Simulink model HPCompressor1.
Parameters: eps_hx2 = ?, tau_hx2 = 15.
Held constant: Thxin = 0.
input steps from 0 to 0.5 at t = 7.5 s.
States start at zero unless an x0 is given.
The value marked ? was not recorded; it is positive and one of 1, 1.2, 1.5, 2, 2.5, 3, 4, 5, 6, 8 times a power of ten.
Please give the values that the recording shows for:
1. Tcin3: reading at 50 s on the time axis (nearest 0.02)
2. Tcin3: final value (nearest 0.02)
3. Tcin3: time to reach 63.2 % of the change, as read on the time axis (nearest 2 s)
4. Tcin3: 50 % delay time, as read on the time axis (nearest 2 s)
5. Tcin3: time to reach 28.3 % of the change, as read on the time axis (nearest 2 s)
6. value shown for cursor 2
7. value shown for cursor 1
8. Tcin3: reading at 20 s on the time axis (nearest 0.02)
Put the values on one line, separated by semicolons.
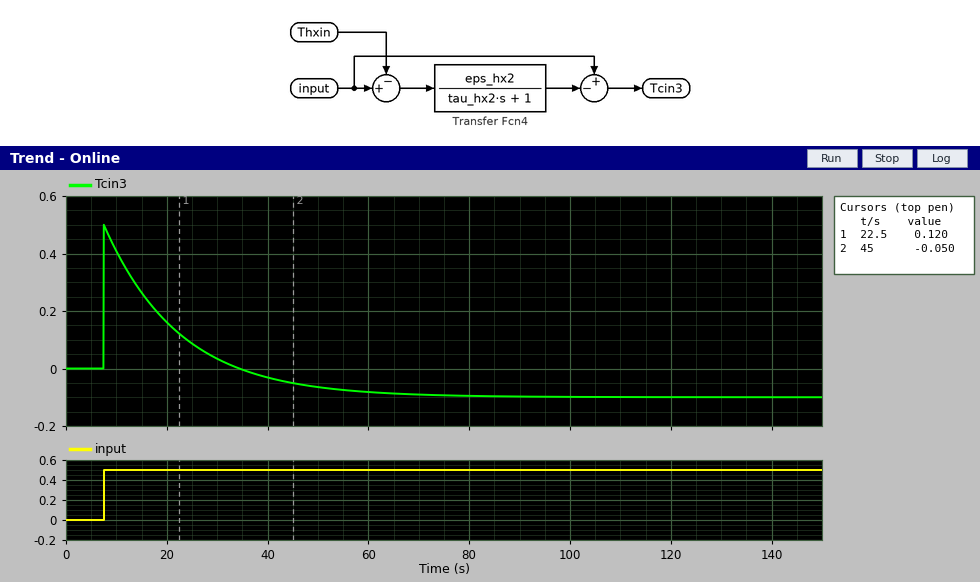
-0.06; -0.10; 50 s; 44 s; 40 s; -0.050; 0.120; 0.16
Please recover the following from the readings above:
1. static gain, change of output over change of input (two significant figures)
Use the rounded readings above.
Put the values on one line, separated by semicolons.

-0.20
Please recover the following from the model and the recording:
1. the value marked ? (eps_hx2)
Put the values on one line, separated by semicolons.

1.2
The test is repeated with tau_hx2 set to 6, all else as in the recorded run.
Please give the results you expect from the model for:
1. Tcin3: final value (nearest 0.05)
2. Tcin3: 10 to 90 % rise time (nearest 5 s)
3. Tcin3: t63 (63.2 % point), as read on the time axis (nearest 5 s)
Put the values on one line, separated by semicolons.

-0.10; 15 s; 25 s
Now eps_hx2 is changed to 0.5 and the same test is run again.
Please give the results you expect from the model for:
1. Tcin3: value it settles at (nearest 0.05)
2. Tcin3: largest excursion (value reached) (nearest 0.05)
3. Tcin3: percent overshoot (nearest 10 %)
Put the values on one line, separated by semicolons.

0.25; 0.50; 100 %
